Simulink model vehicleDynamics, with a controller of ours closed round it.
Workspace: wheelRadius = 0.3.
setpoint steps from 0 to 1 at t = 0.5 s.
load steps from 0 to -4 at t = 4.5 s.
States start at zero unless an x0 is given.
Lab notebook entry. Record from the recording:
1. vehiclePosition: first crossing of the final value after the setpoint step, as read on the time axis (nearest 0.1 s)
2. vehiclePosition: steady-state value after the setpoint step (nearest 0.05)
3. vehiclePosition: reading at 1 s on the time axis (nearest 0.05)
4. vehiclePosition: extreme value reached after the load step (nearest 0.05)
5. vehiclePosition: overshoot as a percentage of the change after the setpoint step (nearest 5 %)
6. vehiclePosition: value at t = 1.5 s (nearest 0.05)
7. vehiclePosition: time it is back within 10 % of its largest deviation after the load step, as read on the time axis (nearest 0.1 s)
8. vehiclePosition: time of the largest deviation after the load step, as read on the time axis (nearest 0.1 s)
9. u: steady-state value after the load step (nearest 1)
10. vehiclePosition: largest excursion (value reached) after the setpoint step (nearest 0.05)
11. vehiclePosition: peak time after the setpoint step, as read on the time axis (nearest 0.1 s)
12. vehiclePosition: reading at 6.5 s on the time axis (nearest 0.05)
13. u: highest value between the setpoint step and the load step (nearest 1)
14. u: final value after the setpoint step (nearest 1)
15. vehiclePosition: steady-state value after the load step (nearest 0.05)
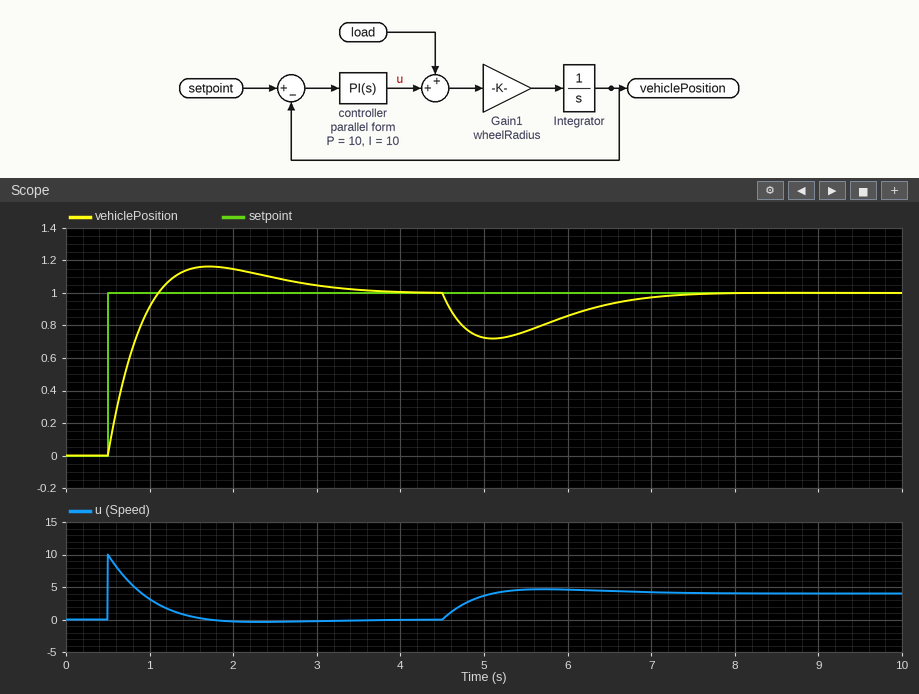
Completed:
1.1 s
1.00
0.90
0.70
15 %
1.15
7.0 s
5.1 s
4
1.15
1.7 s
0.95
10
0
1.00
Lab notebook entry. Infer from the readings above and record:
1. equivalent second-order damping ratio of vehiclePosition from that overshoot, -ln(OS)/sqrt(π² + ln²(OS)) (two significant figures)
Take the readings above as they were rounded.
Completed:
0.52
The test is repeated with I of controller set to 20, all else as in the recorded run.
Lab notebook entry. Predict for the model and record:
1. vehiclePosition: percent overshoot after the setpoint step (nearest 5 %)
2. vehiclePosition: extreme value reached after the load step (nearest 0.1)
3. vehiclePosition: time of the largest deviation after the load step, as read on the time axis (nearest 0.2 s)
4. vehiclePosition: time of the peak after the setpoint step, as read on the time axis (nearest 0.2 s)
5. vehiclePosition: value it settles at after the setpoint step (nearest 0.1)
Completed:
25 %
0.8
5.0 s
1.4 s
1.0
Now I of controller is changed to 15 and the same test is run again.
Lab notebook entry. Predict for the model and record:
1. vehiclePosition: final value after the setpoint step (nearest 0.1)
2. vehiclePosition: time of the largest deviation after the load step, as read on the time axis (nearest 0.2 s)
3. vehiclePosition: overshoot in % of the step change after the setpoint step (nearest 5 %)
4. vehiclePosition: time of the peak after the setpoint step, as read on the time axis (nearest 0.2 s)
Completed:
1.0
5.0 s
20 %
1.6 s
